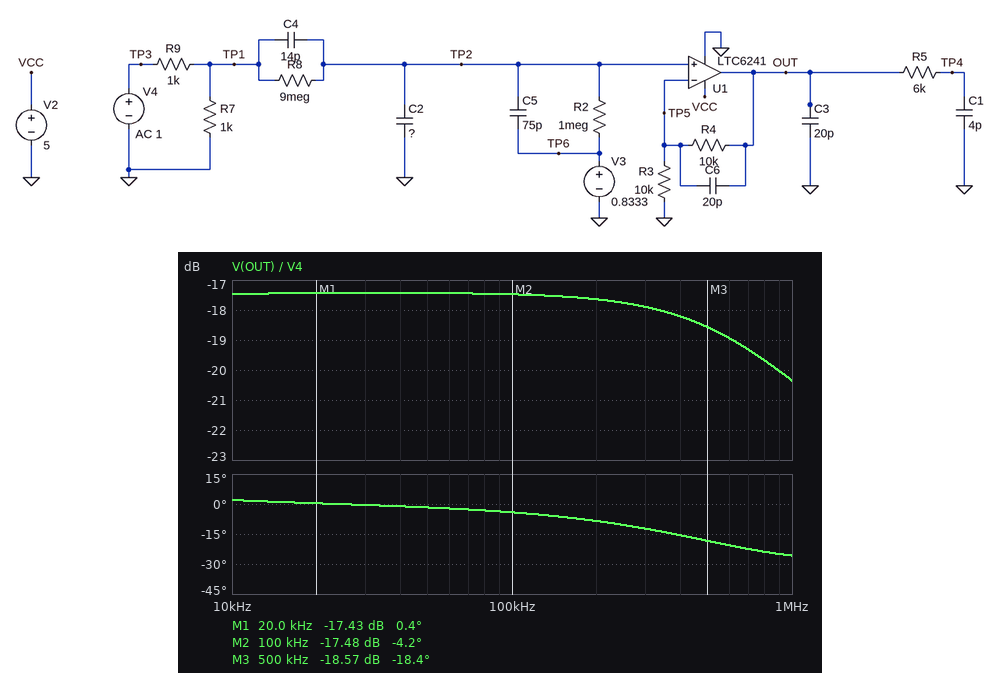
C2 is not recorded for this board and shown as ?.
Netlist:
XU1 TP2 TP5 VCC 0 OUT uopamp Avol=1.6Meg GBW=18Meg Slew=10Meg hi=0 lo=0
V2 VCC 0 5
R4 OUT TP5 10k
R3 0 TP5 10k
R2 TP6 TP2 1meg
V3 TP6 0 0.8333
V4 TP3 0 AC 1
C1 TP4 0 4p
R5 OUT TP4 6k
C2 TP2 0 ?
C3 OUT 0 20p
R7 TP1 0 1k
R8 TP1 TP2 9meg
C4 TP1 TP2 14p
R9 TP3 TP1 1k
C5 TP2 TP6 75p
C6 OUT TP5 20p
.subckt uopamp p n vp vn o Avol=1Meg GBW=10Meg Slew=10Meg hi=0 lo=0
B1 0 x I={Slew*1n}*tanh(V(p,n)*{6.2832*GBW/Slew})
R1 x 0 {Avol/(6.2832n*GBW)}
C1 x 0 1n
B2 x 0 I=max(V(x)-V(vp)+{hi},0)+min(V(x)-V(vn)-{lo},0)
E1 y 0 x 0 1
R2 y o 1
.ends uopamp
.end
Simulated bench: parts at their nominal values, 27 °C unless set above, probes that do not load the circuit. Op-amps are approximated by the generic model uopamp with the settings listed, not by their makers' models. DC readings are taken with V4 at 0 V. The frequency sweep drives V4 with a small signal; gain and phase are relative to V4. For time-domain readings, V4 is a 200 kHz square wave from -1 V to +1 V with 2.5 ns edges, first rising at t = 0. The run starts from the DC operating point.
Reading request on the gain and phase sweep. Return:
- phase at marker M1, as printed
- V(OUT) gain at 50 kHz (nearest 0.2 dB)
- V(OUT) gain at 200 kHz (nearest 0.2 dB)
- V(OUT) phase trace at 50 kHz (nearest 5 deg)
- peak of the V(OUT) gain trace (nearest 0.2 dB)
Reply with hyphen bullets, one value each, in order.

- 0.4 deg
- -17.4 dB
- -17.6 dB
- 0 deg
- -17.4 dB
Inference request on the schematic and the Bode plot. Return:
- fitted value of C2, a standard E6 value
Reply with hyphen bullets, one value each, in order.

- 15 pF
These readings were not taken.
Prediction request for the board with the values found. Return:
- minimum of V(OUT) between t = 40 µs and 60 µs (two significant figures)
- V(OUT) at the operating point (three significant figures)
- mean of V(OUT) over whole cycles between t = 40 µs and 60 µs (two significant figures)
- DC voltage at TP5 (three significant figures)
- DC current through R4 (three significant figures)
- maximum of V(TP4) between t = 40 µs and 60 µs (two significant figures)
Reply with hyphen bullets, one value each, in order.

- 1.4 V
- 1.50 V
- 1.5 V
- 750 mV
- 75.0 µA
- 1.7 V
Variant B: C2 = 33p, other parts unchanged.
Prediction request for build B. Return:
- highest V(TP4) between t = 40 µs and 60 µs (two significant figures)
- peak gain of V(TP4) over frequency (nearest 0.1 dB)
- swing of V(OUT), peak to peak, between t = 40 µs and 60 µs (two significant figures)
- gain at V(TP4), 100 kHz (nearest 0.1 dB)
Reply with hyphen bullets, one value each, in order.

- 1.6 V
- -18.8 dB
- 230 mV
- -18.9 dB
